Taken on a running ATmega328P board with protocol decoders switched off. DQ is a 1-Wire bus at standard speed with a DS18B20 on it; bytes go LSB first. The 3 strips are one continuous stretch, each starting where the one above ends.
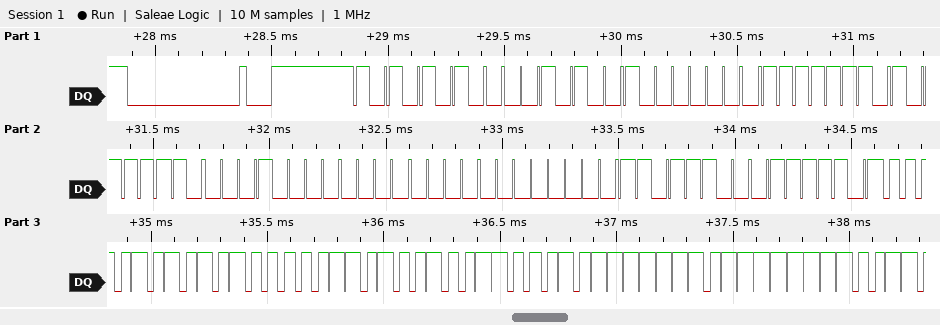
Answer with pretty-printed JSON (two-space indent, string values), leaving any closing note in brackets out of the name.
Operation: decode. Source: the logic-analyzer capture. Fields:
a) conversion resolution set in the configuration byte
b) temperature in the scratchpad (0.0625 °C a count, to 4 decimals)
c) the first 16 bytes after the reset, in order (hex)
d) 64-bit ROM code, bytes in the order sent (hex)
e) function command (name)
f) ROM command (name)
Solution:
{
  "conversion resolution set in the configuration byte": "12 bits",
  "temperature in the scratchpad": "85.0000 °C",
  "the first 16 bytes after the reset, in order": "55 28 01 7F 7D 08 00 00 3B BE 50 05 4B 46 7F FF",
  "64-bit ROM code, bytes in the order sent": "28 01 7F 7D 08 00 00 3B",
  "function command": "Read Scratchpad",
  "ROM command": "Match ROM"
}
